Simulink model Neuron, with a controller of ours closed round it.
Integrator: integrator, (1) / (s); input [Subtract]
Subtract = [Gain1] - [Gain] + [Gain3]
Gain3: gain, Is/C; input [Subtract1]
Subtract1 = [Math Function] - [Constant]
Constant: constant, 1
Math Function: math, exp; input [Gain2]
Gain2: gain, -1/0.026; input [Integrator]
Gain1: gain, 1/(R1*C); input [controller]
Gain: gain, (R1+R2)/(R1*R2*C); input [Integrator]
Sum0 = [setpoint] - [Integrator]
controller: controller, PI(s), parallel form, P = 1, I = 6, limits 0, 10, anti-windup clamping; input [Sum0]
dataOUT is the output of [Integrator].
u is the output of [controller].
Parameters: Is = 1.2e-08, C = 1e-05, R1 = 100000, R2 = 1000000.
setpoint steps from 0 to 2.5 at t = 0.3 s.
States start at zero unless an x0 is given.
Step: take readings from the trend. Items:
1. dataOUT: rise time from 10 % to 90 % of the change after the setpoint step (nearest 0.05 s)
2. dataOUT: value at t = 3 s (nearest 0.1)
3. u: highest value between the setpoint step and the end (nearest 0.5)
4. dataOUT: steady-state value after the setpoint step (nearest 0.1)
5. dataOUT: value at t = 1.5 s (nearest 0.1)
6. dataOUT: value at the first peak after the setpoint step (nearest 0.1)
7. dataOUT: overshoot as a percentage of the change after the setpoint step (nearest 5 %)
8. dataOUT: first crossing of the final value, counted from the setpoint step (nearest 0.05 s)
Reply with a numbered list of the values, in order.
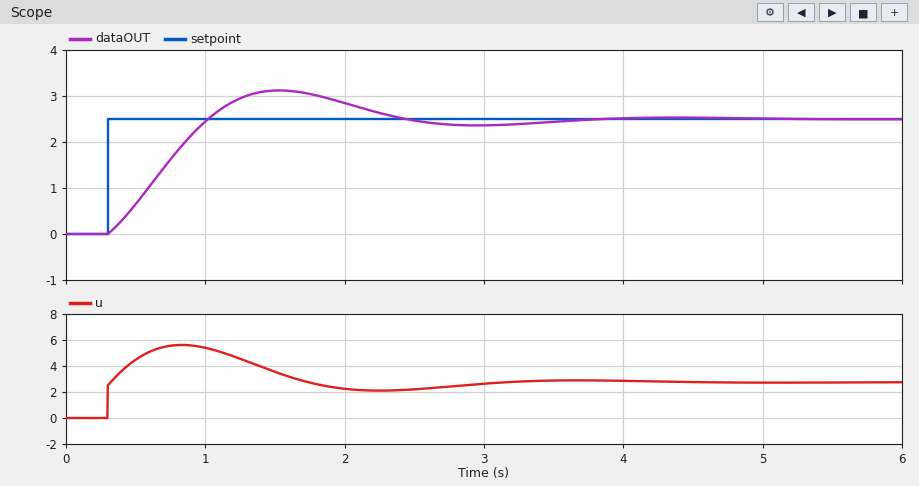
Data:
1. 0.55 s
2. 2.4
3. 5.5
4. 2.5
5. 3.1
6. 3.1
7. 25 %
8. 0.70 s
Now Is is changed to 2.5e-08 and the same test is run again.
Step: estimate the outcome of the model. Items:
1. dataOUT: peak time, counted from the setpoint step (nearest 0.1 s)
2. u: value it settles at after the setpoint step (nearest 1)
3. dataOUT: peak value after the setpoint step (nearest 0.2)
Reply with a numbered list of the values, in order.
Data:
1. 1.2 s
2. 3
3. 3.2
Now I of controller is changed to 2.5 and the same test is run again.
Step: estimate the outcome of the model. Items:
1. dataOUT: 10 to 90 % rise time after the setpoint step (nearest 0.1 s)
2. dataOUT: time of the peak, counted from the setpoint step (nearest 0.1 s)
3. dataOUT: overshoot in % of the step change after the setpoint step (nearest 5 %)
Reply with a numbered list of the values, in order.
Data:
1. 1.0 s
2. 2.1 s
3. 10 %
